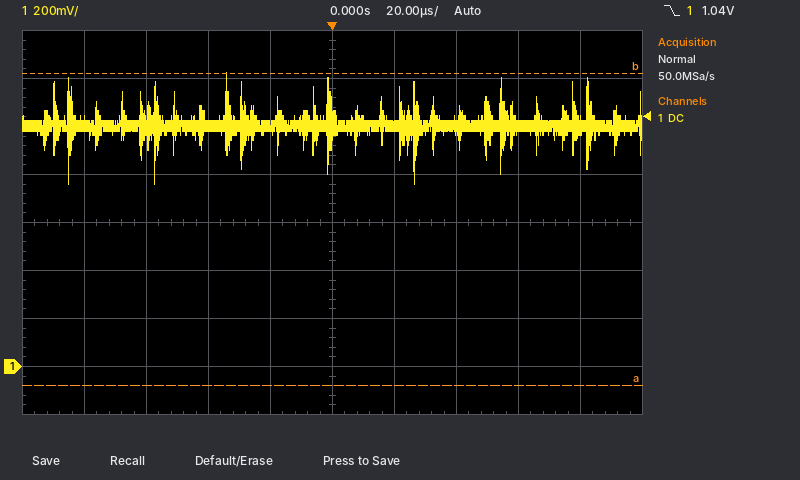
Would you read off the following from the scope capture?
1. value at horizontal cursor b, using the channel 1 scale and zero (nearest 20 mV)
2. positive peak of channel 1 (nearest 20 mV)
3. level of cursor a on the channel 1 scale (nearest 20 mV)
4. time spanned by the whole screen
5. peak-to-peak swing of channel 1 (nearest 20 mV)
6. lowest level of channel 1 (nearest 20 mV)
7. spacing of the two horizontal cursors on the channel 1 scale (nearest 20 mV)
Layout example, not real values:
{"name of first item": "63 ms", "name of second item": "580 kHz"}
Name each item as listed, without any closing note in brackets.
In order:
{"value at horizontal cursor b, using the channel 1 scale and zero": "1.22 V", "positive peak of channel 1": "1.22 V", "level of cursor a on the channel 1 scale": "-80 mV", "time spanned by the whole screen": "200 µs", "peak-to-peak swing of channel 1": "460 mV", "lowest level of channel 1": "760 mV", "spacing of the two horizontal cursors on the channel 1 scale": "1.30 V"}
